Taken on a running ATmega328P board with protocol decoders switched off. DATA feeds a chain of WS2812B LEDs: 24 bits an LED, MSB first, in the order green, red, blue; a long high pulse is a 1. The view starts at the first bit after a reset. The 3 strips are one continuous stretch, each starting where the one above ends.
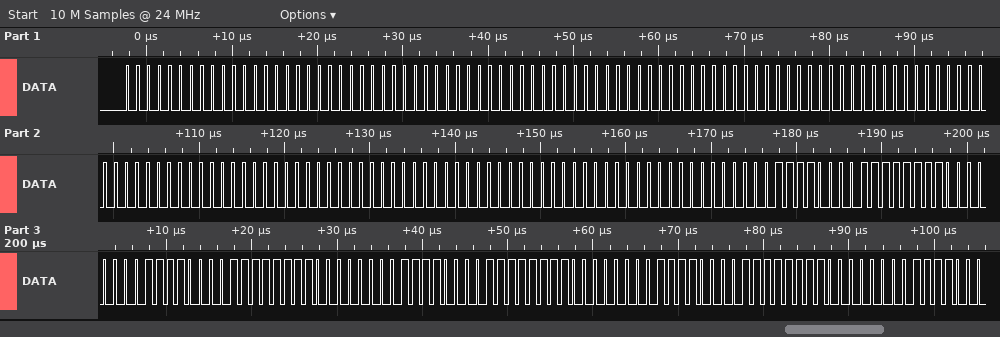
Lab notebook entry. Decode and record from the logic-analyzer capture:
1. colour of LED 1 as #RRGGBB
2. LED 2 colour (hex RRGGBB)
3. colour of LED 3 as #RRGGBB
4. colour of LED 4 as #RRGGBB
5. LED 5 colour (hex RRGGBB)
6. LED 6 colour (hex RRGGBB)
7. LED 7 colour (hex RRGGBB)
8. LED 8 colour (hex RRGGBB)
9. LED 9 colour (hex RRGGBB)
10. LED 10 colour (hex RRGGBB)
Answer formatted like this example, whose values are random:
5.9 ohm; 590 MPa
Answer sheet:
#000000; #000000; #000000; #000000; #000000; #000000; #FFF000; #FFF000; #FFF000; #FFF000
